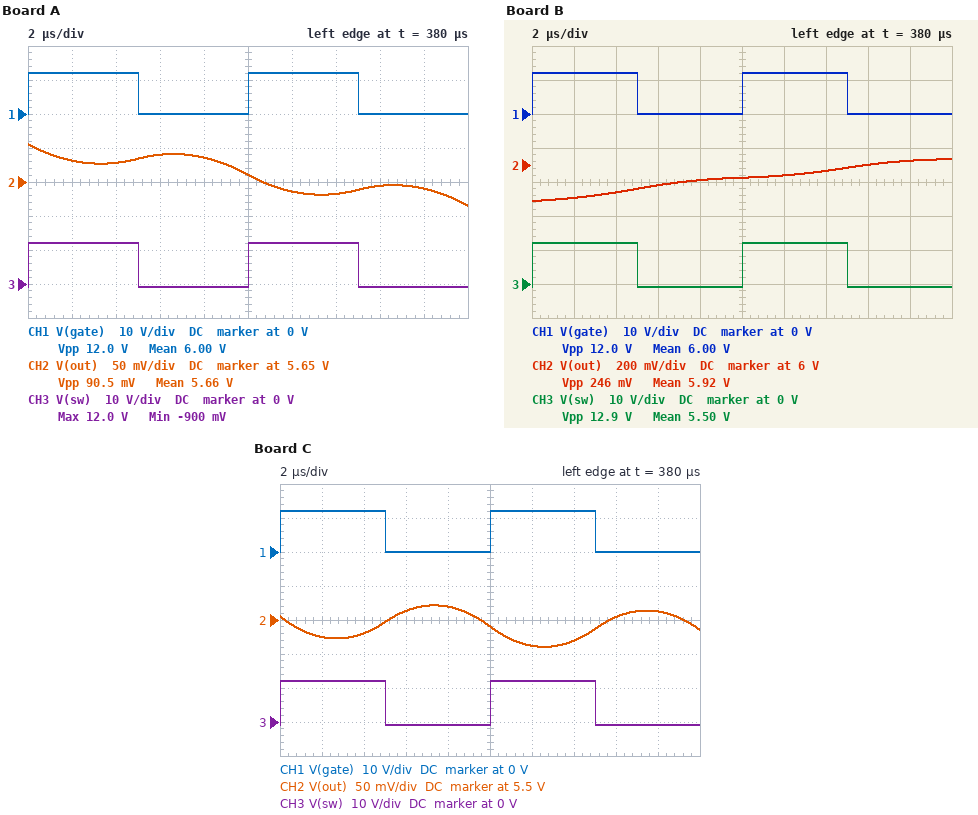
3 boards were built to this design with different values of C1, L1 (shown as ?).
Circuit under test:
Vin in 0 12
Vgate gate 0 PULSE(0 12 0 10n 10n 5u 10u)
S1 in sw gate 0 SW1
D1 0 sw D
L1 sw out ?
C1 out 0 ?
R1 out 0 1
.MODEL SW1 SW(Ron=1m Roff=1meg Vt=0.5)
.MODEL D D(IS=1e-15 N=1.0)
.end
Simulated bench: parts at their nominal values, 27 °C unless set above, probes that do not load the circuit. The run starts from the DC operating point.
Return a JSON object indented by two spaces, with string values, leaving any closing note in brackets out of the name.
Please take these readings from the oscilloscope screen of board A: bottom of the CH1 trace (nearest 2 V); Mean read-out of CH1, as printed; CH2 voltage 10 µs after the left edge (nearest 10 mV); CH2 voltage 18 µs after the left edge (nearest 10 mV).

{
  "bottom of the CH1 trace": "0 V",
  "Mean read-out of CH1, as printed": "6.00 V",
  "CH2 voltage 10 µs after the left edge": "5.66 V",
  "CH2 voltage 18 µs after the left edge": "5.64 V"
}
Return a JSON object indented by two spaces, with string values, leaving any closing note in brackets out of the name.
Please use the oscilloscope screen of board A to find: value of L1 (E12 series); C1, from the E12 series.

{
  "value of L1": "22 µH",
  "C1, from the E12 series": "56 µF"
}
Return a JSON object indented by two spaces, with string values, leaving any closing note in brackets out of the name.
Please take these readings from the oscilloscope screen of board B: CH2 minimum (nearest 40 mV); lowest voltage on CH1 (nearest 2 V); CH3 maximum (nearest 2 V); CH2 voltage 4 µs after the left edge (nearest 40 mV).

{
  "CH2 minimum": "5.80 V",
  "lowest voltage on CH1": "0 V",
  "CH3 maximum": "12 V",
  "CH2 voltage 4 µs after the left edge": "5.84 V"
}
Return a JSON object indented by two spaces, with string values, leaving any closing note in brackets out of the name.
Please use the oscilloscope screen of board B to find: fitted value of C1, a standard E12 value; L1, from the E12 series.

{
  "fitted value of C1, a standard E12 value": "150 µF",
  "L1, from the E12 series": "12 µH"
}
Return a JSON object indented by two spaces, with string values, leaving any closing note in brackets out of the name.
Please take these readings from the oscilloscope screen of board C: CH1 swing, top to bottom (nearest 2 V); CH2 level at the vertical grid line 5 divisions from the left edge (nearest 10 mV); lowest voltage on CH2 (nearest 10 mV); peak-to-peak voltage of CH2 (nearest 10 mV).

{
  "CH1 swing, top to bottom": "12 V",
  "CH2 level at the vertical grid line 5 divisions from the left edge": "5.49 V",
  "lowest voltage on CH2": "5.46 V",
  "peak-to-peak voltage of CH2": "60 mV"
}
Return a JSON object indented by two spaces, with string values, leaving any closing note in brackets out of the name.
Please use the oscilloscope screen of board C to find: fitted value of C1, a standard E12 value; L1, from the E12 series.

{
  "fitted value of C1, a standard E12 value": "220 µF",
  "L1, from the E12 series": "3.3 µH"
}
